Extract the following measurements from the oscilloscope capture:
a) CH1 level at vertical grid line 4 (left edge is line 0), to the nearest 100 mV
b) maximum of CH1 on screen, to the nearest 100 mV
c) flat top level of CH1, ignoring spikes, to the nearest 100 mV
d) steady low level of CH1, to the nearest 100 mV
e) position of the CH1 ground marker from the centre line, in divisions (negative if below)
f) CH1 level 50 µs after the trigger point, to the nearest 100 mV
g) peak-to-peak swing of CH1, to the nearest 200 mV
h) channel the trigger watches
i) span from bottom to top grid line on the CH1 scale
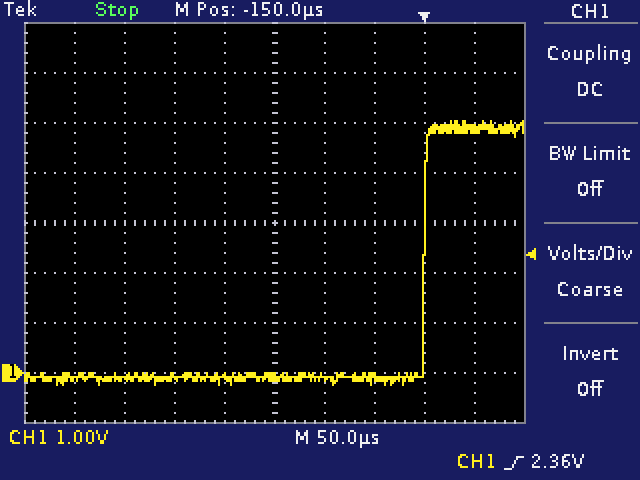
-100 mV
5.0 V
4.9 V
-100 mV
-3.0 div
4.9 V
5.2 V
CH1
8 V
